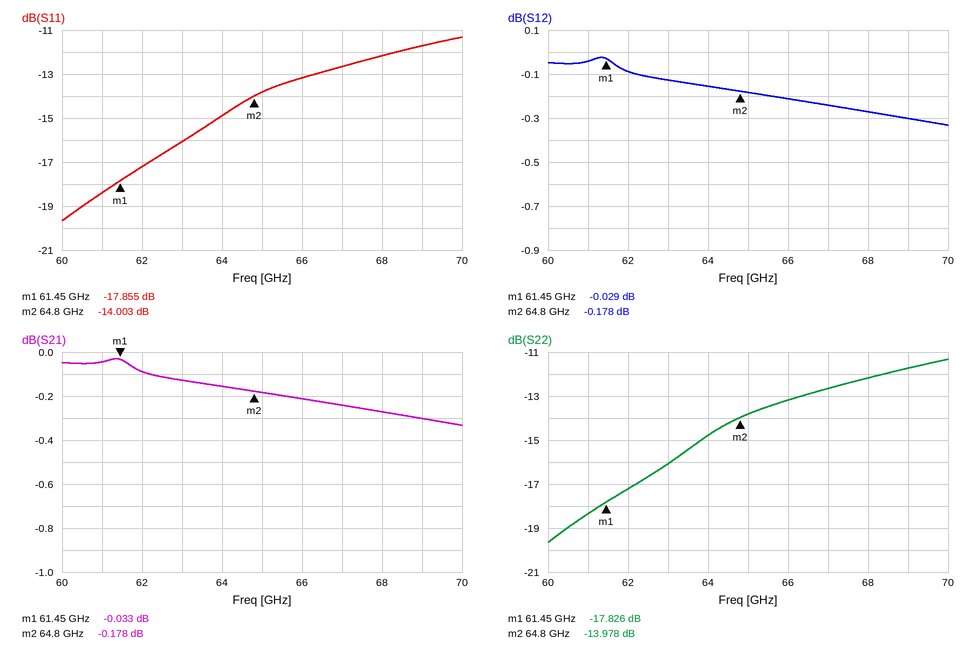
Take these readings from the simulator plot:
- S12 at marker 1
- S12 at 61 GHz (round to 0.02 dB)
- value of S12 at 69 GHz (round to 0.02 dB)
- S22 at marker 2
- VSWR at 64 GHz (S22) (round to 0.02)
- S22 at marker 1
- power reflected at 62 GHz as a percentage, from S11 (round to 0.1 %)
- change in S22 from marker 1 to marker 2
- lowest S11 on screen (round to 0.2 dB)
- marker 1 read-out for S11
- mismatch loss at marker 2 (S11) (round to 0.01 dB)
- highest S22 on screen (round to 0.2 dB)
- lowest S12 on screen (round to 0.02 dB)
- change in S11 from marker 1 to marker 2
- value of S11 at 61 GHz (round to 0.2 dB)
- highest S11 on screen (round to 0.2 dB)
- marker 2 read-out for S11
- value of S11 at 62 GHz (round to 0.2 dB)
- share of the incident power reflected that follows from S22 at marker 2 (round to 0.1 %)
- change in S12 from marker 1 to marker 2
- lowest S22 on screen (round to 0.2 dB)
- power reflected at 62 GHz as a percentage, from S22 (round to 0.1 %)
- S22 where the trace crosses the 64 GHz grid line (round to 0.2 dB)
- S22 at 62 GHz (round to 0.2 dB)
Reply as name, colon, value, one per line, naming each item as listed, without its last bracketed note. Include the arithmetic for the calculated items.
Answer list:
S12 at marker 1: -0.029 dB
S12 at 61 GHz: -0.04 dB
value of S12 at 69 GHz: -0.30 dB
S22 at marker 2: -13.978 dB
VSWR at 64 GHz (S22): |Γ| = 10^(-14.8/20) = 0.1820; VSWR = (1 + 0.1820)/(1 − 0.1820) ≈ 1.44
S22 at marker 1: -17.826 dB
power reflected at 62 GHz as a percentage, from S11: 10^(-17.2/10) ≈ 1.9 %
change in S22 from marker 1 to marker 2: -13.978 − (-17.826) = 3.848 dB
lowest S11 on screen: -19.6 dB
marker 1 read-out for S11: -17.855 dB
mismatch loss at marker 2 (S11): −10 log10(1 − 10^(-14.003/10)) ≈ 0.18 dB
highest S22 on screen: -11.4 dB
lowest S12 on screen: -0.34 dB
change in S11 from marker 1 to marker 2: -14.003 − (-17.855) = 3.852 dB
value of S11 at 61 GHz: -18.4 dB
highest S11 on screen: -11.4 dB
marker 2 read-out for S11: -14.003 dB
value of S11 at 62 GHz: -17.2 dB
share of the incident power reflected that follows from S22 at marker 2: 10^(-13.978/10) ≈ 4.0 %
change in S12 from marker 1 to marker 2: -0.178 − (-0.029) = -0.149 dB
lowest S22 on screen: -19.6 dB
power reflected at 62 GHz as a percentage, from S22: 10^(-17.2/10) ≈ 1.9 %
S22 where the trace crosses the 64 GHz grid line: -14.8 dB
S22 at 62 GHz: -17.2 dB
